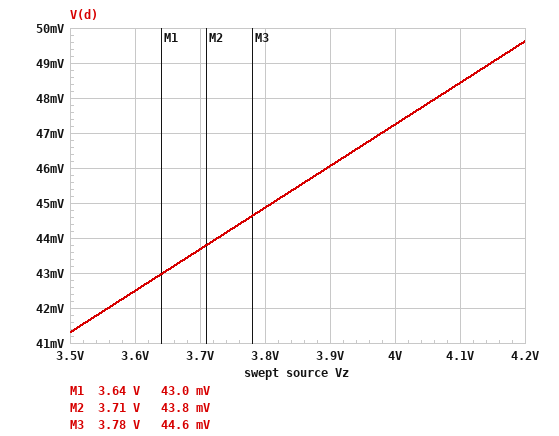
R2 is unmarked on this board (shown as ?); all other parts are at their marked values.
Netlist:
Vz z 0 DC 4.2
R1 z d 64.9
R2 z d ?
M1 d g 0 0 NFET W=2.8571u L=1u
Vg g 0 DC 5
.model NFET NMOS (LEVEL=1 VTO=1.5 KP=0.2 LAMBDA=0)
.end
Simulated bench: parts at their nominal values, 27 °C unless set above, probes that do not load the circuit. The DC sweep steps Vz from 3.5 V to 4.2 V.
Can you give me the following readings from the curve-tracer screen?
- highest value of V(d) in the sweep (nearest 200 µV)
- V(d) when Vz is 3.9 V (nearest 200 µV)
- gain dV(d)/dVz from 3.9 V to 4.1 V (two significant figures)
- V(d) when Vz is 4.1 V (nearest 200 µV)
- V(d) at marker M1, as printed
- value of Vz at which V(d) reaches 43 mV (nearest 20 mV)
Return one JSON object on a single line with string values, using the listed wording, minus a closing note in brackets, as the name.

{"highest value of V(d) in the sweep": "49.6 mV", "V(d) when Vz is 3.9 V": "46.0 mV", "gain dV(d)/dVz from 3.9 V to 4.1 V": "0.012 V/V", "V(d) when Vz is 4.1 V": "48.4 mV", "V(d) at marker M1, as printed": "43.0 mV", "value of Vz at which V(d) reaches 43 mV": "3.64 V"}
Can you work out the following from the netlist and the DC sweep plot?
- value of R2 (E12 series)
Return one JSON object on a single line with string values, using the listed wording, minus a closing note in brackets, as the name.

{"value of R2": "120 Ω"}
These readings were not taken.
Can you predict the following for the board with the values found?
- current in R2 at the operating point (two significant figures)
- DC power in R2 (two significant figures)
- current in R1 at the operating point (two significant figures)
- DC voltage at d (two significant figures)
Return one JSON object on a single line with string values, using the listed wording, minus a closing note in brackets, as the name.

{"current in R2 at the operating point": "35 mA", "DC power in R2": "140 mW", "current in R1 at the operating point": "64 mA", "DC voltage at d": "50 mV"}
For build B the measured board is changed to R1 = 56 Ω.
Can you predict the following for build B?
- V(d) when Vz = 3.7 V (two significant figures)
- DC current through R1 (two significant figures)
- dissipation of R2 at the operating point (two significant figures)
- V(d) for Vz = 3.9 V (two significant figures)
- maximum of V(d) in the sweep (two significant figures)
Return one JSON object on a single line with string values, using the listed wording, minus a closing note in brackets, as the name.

{"V(d) when Vz = 3.7 V": "48 mV", "DC current through R1": "74 mA", "dissipation of R2 at the operating point": "140 mW", "V(d) for Vz = 3.9 V": "51 mV", "maximum of V(d) in the sweep": "55 mV"}
